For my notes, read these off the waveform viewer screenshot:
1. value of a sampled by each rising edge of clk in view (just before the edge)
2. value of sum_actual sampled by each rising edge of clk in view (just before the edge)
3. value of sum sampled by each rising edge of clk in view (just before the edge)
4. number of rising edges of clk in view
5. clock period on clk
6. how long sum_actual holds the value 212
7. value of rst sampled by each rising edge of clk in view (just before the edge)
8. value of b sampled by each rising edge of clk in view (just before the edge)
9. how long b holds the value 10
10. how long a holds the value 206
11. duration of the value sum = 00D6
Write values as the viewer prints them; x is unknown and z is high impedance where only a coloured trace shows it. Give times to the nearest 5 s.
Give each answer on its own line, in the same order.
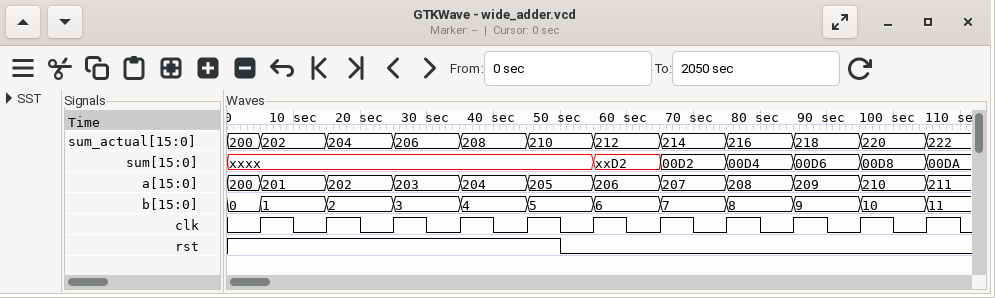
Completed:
200, 201, 202, 203, 204, 205, 206, 207, 208, 209, 210
200, 202, 204, 206, 208, 210, 212, 214, 216, 218, 220
xxxx, xxxx, xxxx, xxxx, xxxx, xxxx, xxD2, 00D2, 00D4, 00D6, 00D8
11
10 s
10 s
1 1 1 1 1 0 0 0 0 0 0
0, 1, 2, 3, 4, 5, 6, 7, 8, 9, 10
10 s
10 s
10 s
